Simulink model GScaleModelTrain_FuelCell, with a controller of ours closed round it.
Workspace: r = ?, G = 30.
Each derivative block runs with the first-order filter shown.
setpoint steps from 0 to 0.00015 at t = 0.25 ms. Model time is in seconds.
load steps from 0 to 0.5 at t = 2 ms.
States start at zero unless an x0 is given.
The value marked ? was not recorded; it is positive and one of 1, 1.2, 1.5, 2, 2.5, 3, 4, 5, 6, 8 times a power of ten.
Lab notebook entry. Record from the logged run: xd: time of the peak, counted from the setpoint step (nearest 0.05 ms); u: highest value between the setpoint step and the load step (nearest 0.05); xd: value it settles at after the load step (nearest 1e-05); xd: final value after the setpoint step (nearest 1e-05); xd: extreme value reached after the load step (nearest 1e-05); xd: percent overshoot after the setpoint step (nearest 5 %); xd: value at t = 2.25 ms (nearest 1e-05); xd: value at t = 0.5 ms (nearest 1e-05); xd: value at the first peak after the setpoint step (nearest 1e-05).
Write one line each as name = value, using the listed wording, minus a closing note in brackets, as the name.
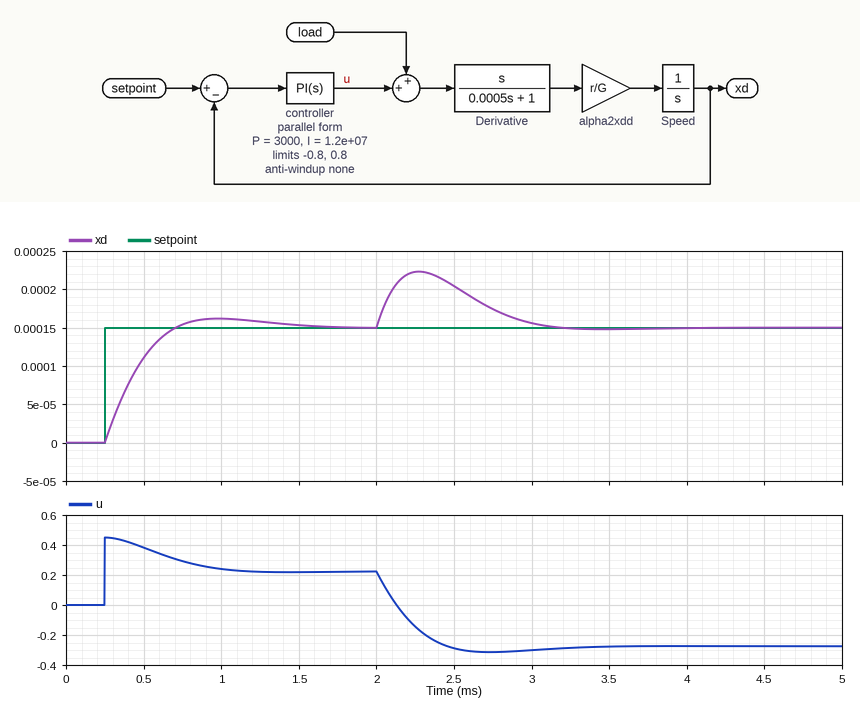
xd: time of the peak, counted from the setpoint step = 0.75 ms
u: highest value between the setpoint step and the load step = 0.45
xd: value it settles at after the load step = 0.00015
xd: final value after the setpoint step = 0.00015
xd: extreme value reached after the load step = 0.00022
xd: percent overshoot after the setpoint step = 10 %
xd: value at t = 2.25 ms = 0.00022
xd: value at t = 0.5 ms = 0.00011
xd: value at the first peak after the setpoint step = 0.00016
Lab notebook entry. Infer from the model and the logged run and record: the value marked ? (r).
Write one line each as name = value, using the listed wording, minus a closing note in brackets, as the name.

the value marked ? = 0.02
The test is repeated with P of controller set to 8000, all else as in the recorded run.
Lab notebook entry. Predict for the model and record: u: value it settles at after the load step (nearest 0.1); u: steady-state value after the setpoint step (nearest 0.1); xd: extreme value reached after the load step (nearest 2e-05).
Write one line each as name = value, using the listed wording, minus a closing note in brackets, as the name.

u: value it settles at after the load step = -0.3
u: steady-state value after the setpoint step = 0.2
xd: extreme value reached after the load step = 0.00020
